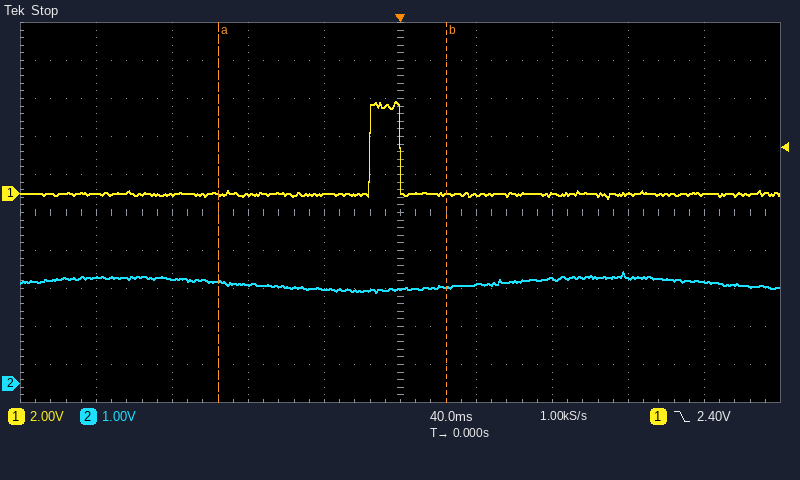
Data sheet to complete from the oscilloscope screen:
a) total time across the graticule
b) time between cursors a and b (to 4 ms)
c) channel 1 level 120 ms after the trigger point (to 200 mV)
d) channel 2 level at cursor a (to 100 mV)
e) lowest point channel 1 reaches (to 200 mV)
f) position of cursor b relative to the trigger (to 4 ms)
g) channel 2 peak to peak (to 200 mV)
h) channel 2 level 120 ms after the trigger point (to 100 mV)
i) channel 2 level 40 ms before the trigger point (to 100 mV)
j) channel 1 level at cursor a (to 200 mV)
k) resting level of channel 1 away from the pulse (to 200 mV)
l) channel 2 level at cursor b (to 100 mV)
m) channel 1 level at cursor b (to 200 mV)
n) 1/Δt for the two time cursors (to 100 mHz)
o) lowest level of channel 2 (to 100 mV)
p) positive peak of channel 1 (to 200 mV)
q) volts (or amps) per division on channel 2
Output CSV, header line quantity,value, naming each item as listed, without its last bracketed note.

quantity,value
total time across the graticule,400 ms
time between cursors a and b,120 ms
channel 1 level 120 ms after the trigger point,0.0 V
channel 2 level at cursor a,2.7 V
lowest point channel 1 reaches,-200 mV
position of cursor b relative to the trigger,+24 ms
channel 2 peak to peak,600 mV
channel 2 level 120 ms after the trigger point,2.8 V
channel 2 level 40 ms before the trigger point,2.5 V
channel 1 level at cursor a,0.0 V
resting level of channel 1 away from the pulse,0.0 V
channel 2 level at cursor b,2.5 V
channel 1 level at cursor b,0.0 V
1/Δt for the two time cursors,8.3 Hz
lowest level of channel 2,2.4 V
positive peak of channel 1,4.8 V
volts (or amps) per division on channel 2,1 V
